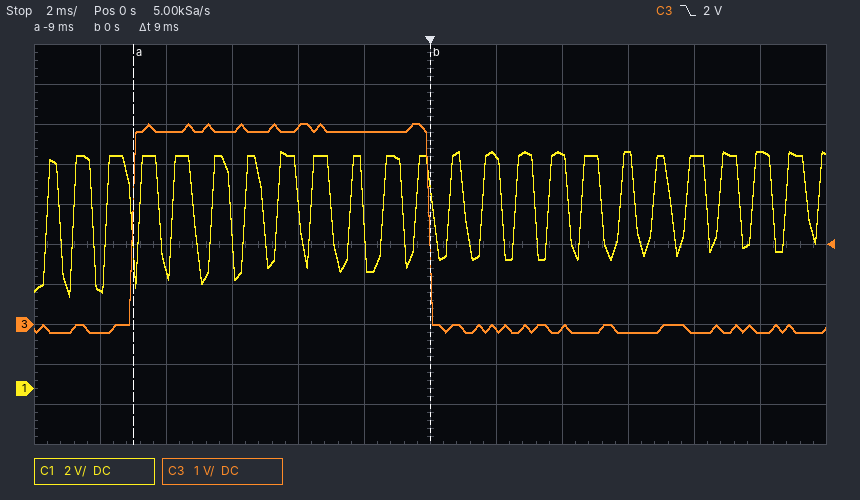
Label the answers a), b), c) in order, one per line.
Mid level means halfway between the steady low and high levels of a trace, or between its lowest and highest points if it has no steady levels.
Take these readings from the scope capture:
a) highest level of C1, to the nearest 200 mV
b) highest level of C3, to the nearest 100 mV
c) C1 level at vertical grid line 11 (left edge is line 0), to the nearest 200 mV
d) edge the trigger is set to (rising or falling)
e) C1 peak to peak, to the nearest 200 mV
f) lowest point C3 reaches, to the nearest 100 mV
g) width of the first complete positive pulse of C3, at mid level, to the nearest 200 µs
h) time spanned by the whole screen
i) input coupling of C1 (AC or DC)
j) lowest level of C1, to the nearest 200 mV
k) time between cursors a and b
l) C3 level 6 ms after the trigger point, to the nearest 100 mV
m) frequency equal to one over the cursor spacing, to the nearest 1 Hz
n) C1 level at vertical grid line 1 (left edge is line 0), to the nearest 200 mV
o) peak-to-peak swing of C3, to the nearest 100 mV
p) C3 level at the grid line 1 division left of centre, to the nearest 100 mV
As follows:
a) 11.8 V
b) 5.0 V
c) 11.8 V
d) falling
e) 7.2 V
f) -200 mV
g) 9.0 ms
h) 24 ms
i) DC
j) 4.6 V
k) 9 ms
l) -200 mV
m) 111 Hz
n) 5.0 V
o) 5.2 V
p) 4.8 V
